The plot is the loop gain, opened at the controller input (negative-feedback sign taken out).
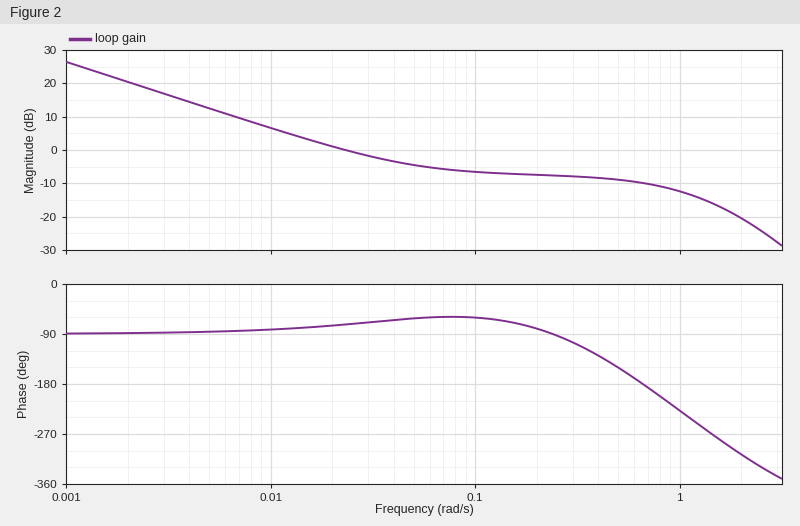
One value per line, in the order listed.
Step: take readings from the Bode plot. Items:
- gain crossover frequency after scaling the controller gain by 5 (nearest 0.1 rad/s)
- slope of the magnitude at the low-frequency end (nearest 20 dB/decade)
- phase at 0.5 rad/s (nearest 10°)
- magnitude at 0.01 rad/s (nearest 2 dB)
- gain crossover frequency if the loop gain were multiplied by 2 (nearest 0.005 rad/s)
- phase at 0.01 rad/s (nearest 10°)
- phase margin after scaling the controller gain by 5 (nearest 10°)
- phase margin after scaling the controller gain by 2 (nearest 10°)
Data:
1.2 rad/s
-20 dB/decade
-150°
6 dB
0.080 rad/s
-80°
-70°
120°
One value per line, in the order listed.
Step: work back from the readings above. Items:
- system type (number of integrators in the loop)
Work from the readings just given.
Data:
1
